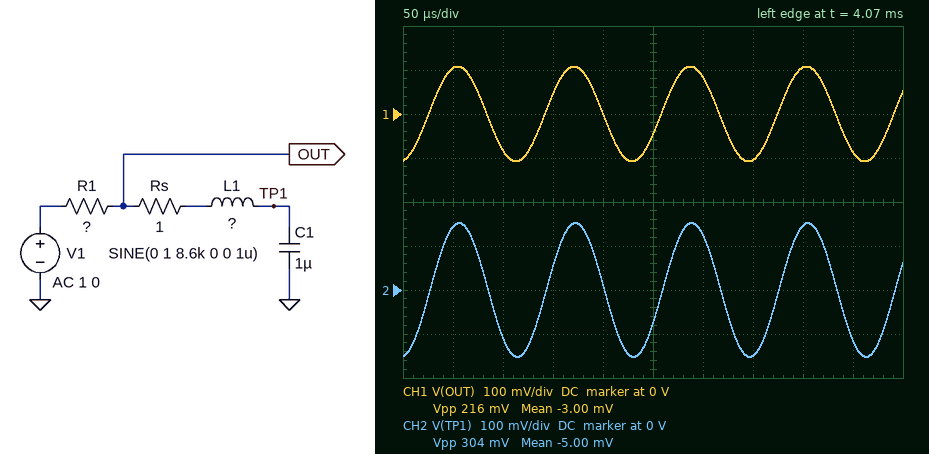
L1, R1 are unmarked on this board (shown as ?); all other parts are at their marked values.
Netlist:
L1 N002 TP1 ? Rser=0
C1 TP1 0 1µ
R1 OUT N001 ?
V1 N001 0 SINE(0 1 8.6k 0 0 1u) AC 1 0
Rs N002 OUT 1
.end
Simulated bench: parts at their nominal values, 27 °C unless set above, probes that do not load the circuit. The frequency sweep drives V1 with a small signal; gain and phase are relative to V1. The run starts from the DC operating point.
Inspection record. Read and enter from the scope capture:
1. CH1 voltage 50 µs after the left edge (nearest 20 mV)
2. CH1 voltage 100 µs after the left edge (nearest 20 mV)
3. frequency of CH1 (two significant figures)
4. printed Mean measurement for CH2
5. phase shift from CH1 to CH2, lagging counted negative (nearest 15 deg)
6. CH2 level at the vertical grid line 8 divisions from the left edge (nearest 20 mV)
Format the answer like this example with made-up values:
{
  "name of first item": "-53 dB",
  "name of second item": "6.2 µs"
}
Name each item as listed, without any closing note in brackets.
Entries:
{
  "CH1 voltage 50 µs after the left edge": "100 mV",
  "CH1 voltage 100 µs after the left edge": "-80 mV",
  "frequency of CH1": "8.6 kHz",
  "printed Mean measurement for CH2": "-5.00 mV",
  "phase shift from CH1 to CH2, lagging counted negative": "0 deg",
  "CH2 level at the vertical grid line 8 divisions from the left edge": "140 mV"
}
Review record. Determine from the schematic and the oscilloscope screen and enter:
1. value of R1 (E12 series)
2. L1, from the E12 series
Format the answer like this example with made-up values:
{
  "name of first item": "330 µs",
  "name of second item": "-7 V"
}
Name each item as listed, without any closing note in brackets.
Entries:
{
  "value of R1": "120 Ω",
  "L1, from the E12 series": "100 µH"
}
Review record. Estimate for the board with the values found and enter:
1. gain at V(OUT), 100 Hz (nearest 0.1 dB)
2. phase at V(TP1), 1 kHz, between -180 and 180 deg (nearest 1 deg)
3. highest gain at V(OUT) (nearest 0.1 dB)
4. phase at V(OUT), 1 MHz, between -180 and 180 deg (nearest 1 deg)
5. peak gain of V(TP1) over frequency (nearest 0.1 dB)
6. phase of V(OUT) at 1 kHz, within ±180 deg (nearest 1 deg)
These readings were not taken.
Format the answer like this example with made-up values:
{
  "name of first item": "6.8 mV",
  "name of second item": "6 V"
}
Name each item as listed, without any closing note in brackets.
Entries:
{
  "gain at V(OUT), 100 Hz": "0 dB",
  "phase at V(TP1), 1 kHz, between -180 and 180 deg": "-37 deg",
  "highest gain at V(OUT)": "0 dB",
  "phase at V(OUT), 1 MHz, between -180 and 180 deg": "11 deg",
  "peak gain of V(TP1) over frequency": "0 dB",
  "phase of V(OUT) at 1 kHz, within ±180 deg": "-37 deg"
}
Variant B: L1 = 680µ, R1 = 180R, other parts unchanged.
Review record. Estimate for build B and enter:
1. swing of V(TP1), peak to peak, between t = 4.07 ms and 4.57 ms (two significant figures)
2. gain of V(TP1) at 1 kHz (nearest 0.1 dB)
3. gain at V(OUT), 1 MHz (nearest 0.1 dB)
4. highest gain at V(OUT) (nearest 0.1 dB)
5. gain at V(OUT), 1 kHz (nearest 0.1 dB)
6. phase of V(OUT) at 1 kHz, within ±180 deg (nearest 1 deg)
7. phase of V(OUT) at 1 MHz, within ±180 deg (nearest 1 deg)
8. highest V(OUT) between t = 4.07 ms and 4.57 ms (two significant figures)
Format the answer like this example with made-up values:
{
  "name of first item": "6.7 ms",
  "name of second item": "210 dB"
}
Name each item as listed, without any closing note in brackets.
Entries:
{
  "swing of V(TP1), peak to peak, between t = 4.07 ms and 4.57 ms": "200 mV",
  "gain of V(TP1) at 1 kHz": "-3.5 dB",
  "gain at V(OUT), 1 MHz": "0 dB",
  "highest gain at V(OUT)": "0 dB",
  "gain at V(OUT), 1 kHz": "-3.7 dB",
  "phase of V(OUT) at 1 kHz, within ±180 deg": "-49 deg",
  "phase of V(OUT) at 1 MHz, within ±180 deg": "2 deg",
  "highest V(OUT) between t = 4.07 ms and 4.57 ms": "100 mV"
}
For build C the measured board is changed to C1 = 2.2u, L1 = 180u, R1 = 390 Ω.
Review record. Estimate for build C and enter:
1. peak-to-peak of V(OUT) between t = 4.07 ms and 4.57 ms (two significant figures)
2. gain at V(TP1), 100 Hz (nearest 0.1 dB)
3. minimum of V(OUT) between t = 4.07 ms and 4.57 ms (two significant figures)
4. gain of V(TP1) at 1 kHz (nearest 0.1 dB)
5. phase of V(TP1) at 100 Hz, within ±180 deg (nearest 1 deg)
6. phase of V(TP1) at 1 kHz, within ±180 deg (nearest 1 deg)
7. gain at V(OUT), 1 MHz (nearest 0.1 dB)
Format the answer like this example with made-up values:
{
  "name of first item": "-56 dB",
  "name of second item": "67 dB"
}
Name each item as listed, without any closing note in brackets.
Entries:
{
  "peak-to-peak of V(OUT) between t = 4.07 ms and 4.57 ms": "8.5 mV",
  "gain at V(TP1), 100 Hz": "-1.1 dB",
  "minimum of V(OUT) between t = 4.07 ms and 4.57 ms": "-4.1 mV",
  "gain of V(TP1) at 1 kHz": "-14.8 dB",
  "phase of V(TP1) at 100 Hz, within ±180 deg": "-28 deg",
  "phase of V(TP1) at 1 kHz, within ±180 deg": "-80 deg",
  "gain at V(OUT), 1 MHz": "-0.5 dB"
}
